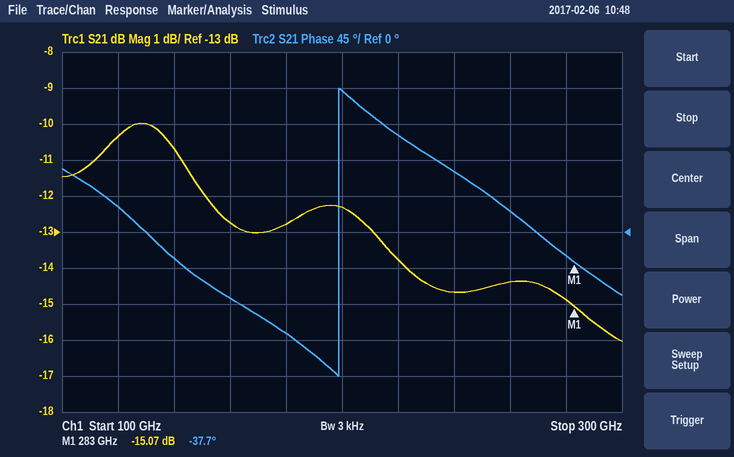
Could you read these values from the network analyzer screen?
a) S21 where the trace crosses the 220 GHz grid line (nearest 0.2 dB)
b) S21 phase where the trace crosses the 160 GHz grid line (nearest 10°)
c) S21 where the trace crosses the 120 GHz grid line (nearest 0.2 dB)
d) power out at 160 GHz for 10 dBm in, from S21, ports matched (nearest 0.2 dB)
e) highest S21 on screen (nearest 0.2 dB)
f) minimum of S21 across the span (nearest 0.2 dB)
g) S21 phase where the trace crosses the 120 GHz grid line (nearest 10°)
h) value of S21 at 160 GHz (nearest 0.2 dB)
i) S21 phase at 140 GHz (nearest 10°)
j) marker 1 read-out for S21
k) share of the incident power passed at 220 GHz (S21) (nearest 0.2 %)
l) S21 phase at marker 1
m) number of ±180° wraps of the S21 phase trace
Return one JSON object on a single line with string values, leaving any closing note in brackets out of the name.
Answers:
{"S21 where the trace crosses the 220 GHz grid line": "-13.8 dB", "S21 phase where the trace crosses the 160 GHz grid line": "-80°", "S21 where the trace crosses the 120 GHz grid line": "-10.4 dB", "power out at 160 GHz for 10 dBm in, from S21, ports matched": "-2.8 dBm", "highest S21 on screen": "-10.0 dB", "minimum of S21 across the span": "-16.0 dB", "S21 phase where the trace crosses the 120 GHz grid line": "30°", "value of S21 at 160 GHz": "-12.8 dB", "S21 phase at 140 GHz": "-30°", "marker 1 read-out for S21": "-15.07 dB", "share of the incident power passed at 220 GHz (S21)": "4.2 %", "S21 phase at marker 1": "-37.7°", "number of ±180° wraps of the S21 phase trace": "1"}
